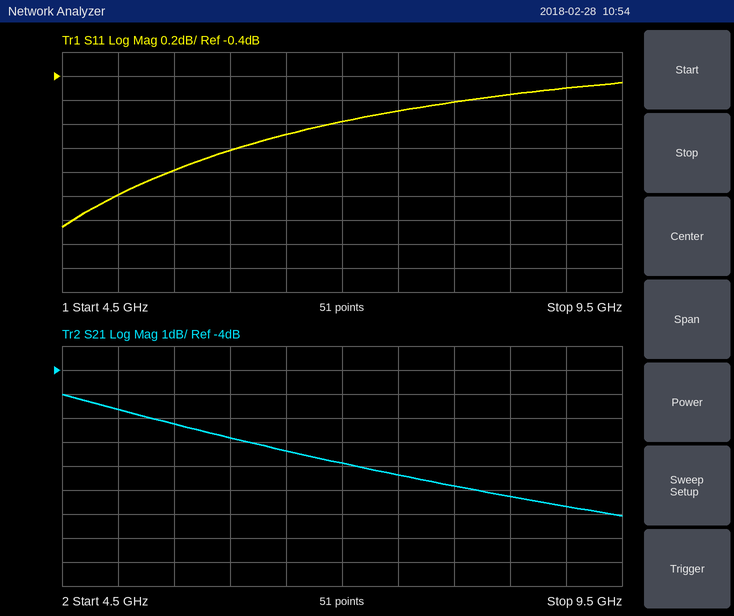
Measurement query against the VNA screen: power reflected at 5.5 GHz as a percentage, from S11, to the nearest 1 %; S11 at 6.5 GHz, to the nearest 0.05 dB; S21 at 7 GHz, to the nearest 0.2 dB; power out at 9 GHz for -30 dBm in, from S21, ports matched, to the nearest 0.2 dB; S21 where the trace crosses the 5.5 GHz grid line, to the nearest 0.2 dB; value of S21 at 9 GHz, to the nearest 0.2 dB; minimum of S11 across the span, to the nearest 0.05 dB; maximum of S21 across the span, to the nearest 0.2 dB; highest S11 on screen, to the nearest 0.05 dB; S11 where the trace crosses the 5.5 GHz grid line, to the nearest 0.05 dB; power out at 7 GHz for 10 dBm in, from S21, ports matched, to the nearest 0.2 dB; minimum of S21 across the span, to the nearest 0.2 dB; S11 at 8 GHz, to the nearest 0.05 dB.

76 %
-0.90 dB
-7.8 dB
-39.6 dBm
-6.2 dB
-9.6 dB
-1.65 dB
-5.0 dB
-0.45 dB
-1.20 dB
2.2 dBm
-10.0 dB
-0.60 dB
